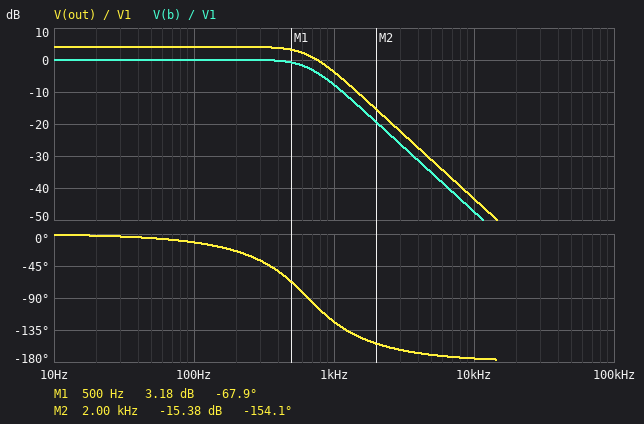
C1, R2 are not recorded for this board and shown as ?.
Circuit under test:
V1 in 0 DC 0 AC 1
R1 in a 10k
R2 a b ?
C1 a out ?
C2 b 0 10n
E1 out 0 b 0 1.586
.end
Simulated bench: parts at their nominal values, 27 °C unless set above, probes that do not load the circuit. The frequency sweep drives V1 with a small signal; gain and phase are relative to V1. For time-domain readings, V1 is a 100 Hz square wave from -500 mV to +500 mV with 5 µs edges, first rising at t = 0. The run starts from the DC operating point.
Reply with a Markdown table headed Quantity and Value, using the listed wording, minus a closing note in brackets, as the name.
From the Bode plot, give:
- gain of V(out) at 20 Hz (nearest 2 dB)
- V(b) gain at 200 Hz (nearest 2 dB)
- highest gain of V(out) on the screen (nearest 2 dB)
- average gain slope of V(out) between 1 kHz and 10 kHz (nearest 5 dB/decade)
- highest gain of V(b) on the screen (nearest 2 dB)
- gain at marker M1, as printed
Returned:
| Quantity | Value |
|---|---|
| gain of V(out) at 20 Hz | 4 dB |
| V(b) gain at 200 Hz | 0 dB |
| highest gain of V(out) on the screen | 4 dB |
| average gain slope of V(out) between 1 kHz and 10 kHz | -40 dB/decade |
| highest gain of V(b) on the screen | 0 dB |
| gain at marker M1, as printed | 3.18 dB |
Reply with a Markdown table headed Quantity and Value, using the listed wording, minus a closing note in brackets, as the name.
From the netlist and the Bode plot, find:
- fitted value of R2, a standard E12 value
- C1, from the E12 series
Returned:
| Quantity | Value |
|---|---|
| fitted value of R2, a standard E12 value | 33 kΩ |
| C1, from the E12 series | 18 nF |
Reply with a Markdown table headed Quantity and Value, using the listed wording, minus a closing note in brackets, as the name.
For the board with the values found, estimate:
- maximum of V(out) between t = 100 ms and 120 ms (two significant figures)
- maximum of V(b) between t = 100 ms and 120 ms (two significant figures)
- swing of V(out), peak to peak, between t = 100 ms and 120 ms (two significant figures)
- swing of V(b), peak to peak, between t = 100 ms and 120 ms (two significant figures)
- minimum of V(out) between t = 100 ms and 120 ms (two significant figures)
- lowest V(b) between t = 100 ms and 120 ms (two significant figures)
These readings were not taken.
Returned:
| Quantity | Value |
|---|---|
| maximum of V(out) between t = 100 ms and 120 ms | 890 mV |
| maximum of V(b) between t = 100 ms and 120 ms | 560 mV |
| swing of V(out), peak to peak, between t = 100 ms and 120 ms | 1.8 V |
| swing of V(b), peak to peak, between t = 100 ms and 120 ms | 1.1 V |
| minimum of V(out) between t = 100 ms and 120 ms | -890 mV |
| lowest V(b) between t = 100 ms and 120 ms | -560 mV |
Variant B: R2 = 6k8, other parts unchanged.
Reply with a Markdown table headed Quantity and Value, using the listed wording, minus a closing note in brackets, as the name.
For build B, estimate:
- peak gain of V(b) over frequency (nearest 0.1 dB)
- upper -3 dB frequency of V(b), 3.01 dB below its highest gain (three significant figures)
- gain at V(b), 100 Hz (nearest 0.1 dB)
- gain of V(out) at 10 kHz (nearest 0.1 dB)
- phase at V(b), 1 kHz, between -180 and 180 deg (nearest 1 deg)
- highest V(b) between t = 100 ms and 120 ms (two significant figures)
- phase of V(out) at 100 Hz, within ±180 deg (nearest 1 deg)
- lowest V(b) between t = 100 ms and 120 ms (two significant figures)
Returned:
| Quantity | Value |
|---|---|
| peak gain of V(b) over frequency | 5.3 dB |
| upper -3 dB frequency of V(b), 3.01 dB below its highest gain | 1.69 kHz |
| gain at V(b), 100 Hz | 0 dB |
| gain of V(out) at 10 kHz | -29.5 dB |
| phase at V(b), 1 kHz, between -180 and 180 deg | -37 deg |
| highest V(b) between t = 100 ms and 120 ms | 900 mV |
| phase of V(out) at 100 Hz, within ±180 deg | -2 deg |
| lowest V(b) between t = 100 ms and 120 ms | -900 mV |
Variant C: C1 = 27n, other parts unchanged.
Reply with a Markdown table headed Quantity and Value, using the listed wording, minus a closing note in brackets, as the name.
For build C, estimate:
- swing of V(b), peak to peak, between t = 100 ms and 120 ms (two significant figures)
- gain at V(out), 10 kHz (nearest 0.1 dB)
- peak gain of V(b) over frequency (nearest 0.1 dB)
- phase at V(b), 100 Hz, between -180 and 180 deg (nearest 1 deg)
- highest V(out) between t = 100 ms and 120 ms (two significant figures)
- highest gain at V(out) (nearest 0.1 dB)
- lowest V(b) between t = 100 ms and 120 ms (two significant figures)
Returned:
| Quantity | Value |
|---|---|
| swing of V(b), peak to peak, between t = 100 ms and 120 ms | 1.4 V |
| gain at V(out), 10 kHz | -46.9 dB |
| peak gain of V(b) over frequency | 1.8 dB |
| phase at V(b), 100 Hz, between -180 and 180 deg | -10 deg |
| highest V(out) between t = 100 ms and 120 ms | 1.1 V |
| highest gain at V(out) | 5.8 dB |
| lowest V(b) between t = 100 ms and 120 ms | -700 mV |
